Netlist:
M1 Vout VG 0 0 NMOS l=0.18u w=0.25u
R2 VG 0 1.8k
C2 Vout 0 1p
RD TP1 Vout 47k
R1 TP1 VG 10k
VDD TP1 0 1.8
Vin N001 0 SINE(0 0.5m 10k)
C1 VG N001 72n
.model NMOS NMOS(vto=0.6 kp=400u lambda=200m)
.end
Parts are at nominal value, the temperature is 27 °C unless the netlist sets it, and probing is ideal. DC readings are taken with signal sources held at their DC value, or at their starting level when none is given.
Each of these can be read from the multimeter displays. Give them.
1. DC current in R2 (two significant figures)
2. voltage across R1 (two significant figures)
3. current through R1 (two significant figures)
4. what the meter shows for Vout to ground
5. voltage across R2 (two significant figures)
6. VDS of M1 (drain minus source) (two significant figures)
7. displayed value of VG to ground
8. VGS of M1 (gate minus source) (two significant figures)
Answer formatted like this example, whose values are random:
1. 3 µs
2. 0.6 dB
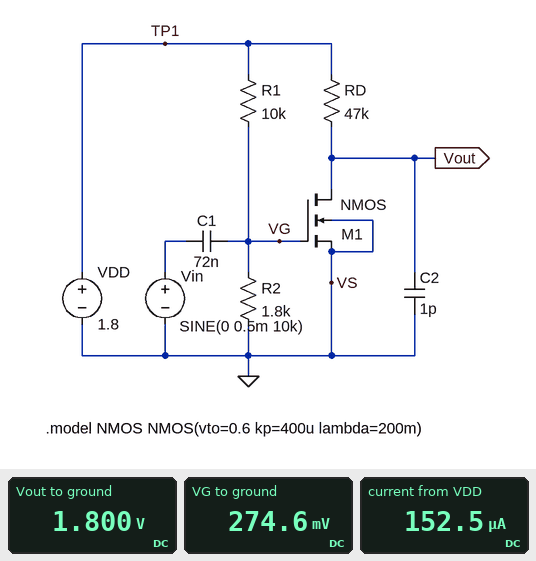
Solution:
1. 150 µA
2. 1.5 V
3. 150 µA
4. 1.800 V
5. 270 mV
6. 1.8 V
7. 274.6 mV
8. 270 mV
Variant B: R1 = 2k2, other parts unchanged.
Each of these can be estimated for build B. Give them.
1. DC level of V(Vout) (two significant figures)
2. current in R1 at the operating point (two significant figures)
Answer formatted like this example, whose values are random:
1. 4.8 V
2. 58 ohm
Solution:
1. 1.1 V
2. 450 µA
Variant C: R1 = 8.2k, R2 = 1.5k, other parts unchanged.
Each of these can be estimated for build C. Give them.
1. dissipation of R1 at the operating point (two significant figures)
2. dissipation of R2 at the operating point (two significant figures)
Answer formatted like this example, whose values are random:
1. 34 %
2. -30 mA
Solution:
1. 280 µW
2. 52 µW
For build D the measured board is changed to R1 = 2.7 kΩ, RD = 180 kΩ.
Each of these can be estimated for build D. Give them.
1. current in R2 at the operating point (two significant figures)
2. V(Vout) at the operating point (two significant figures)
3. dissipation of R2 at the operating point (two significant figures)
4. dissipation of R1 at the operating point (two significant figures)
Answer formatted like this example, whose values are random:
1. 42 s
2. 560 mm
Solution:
1. 400 µA
2. 940 mV
3. 290 µW
4. 430 µW
